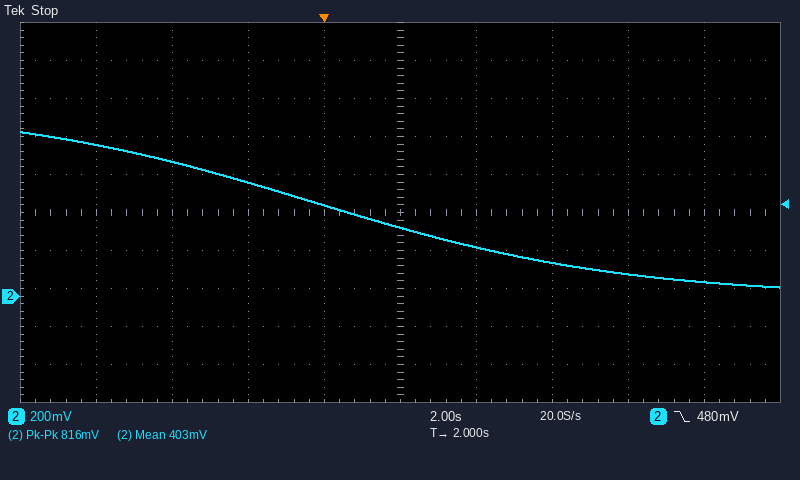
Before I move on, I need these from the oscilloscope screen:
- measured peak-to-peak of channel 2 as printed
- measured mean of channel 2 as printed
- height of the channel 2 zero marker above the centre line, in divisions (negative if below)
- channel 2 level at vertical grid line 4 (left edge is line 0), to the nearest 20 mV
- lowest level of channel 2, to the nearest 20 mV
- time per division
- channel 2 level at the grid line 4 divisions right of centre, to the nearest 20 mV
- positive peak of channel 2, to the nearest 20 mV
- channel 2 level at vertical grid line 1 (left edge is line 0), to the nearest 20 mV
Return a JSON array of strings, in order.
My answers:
["816 mV", "403 mV", "-2.2 div", "480 mV", "40 mV", "2 s", "80 mV", "860 mV", "800 mV"]
